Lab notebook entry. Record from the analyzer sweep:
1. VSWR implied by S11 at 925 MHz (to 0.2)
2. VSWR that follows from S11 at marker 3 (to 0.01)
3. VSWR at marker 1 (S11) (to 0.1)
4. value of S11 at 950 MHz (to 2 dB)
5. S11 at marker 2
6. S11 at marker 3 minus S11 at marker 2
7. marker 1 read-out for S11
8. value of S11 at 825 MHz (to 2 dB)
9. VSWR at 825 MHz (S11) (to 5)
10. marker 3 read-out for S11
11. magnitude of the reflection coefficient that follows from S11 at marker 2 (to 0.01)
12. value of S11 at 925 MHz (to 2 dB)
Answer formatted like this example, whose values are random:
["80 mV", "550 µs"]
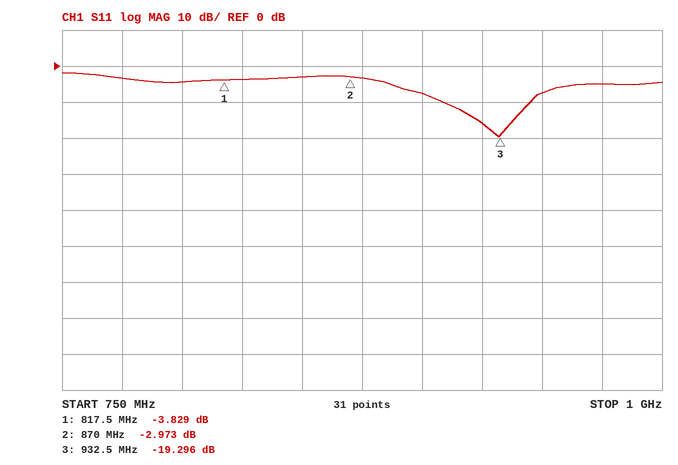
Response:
["1.4", "1.24", "4.6", "-8 dB", "-2.973 dB", "-16.323 dB", "-3.829 dB", "-4 dB", "5", "-19.296 dB", "0.71", "-16 dB"]
